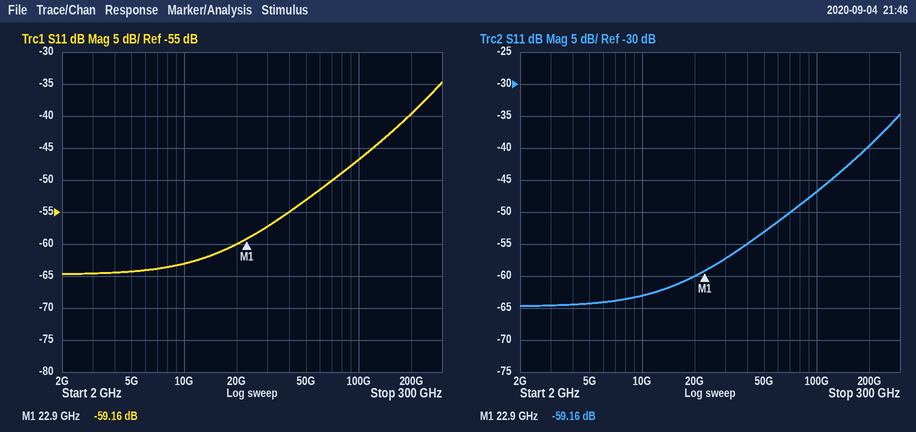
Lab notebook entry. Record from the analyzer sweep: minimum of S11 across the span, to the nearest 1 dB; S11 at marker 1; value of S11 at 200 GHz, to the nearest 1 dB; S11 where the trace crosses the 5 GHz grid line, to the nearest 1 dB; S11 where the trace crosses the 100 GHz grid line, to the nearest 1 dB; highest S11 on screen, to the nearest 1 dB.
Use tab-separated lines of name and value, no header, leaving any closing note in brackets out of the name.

minimum of S11 across the span, to the nearest 1 dB	-65 dB
S11 at marker 1	-59.16 dB
value of S11 at 200 GHz, to the nearest 1 dB	-40 dB
S11 where the trace crosses the 5 GHz grid line, to the nearest 1 dB	-64 dB
S11 where the trace crosses the 100 GHz grid line, to the nearest 1 dB	-47 dB
highest S11 on screen, to the nearest 1 dB	-35 dB
